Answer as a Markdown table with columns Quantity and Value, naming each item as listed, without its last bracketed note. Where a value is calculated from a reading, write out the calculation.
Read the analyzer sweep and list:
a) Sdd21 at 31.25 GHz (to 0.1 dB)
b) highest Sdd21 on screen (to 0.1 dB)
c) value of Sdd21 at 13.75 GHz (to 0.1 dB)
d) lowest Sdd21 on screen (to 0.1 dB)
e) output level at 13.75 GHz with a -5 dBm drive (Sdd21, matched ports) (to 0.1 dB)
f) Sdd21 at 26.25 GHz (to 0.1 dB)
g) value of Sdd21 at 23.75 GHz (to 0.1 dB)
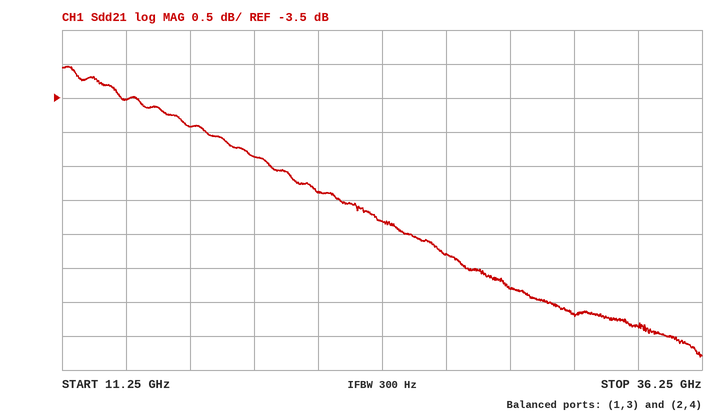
| Quantity | Value |
|---|---|
| Sdd21 at 31.25 GHz | -6.7 dB |
| highest Sdd21 on screen | -3.0 dB |
| value of Sdd21 at 13.75 GHz | -3.5 dB |
| lowest Sdd21 on screen | -7.3 dB |
| output level at 13.75 GHz with a -5 dBm drive (Sdd21, matched ports) | -5 dBm + (-3.5 dB) = -8.5 dBm |
| Sdd21 at 26.25 GHz | -5.8 dB |
| value of Sdd21 at 23.75 GHz | -5.3 dB |
